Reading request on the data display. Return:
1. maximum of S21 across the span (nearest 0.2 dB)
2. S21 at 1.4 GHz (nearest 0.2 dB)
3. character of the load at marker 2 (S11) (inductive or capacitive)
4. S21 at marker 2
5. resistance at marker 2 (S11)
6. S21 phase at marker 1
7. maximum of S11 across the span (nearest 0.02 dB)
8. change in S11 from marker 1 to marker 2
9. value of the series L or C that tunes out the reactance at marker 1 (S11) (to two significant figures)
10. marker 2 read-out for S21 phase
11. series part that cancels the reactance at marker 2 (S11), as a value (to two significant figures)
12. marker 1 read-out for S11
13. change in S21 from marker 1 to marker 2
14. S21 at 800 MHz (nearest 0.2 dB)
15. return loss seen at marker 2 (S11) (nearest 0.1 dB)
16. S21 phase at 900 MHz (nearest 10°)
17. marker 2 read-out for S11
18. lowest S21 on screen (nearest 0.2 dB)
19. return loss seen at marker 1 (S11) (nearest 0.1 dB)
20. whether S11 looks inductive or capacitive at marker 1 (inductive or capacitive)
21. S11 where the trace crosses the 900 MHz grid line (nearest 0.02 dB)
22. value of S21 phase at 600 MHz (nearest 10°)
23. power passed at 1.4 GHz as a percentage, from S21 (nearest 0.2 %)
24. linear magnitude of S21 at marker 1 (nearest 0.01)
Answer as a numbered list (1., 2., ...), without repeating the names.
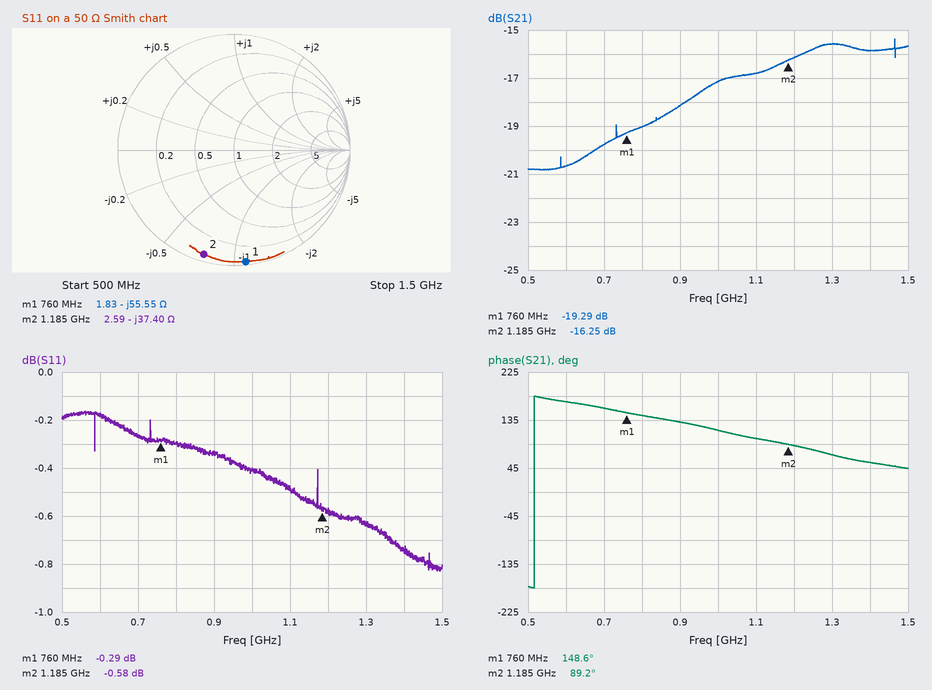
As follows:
1. -15.4 dB
2. -15.8 dB
3. capacitive
4. -16.25 dB
5. 2.59 Ω
6. 148.6°
7. -0.16 dB
8. -0.29 dB
9. 12 nH
10. 89.2°
11. 5.0 nH
12. -0.29 dB
13. 3.04 dB
14. -19.0 dB
15. 0.6 dB
16. 130°
17. -0.58 dB
18. -20.8 dB
19. 0.3 dB
20. capacitive
21. -0.34 dB
22. 170°
23. 2.6 %
24. 0.11
